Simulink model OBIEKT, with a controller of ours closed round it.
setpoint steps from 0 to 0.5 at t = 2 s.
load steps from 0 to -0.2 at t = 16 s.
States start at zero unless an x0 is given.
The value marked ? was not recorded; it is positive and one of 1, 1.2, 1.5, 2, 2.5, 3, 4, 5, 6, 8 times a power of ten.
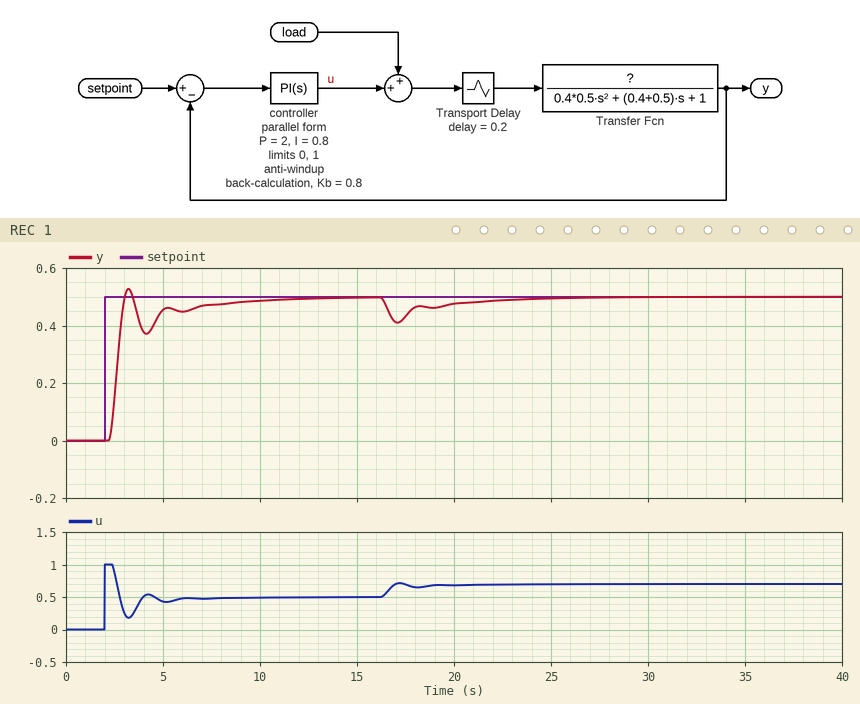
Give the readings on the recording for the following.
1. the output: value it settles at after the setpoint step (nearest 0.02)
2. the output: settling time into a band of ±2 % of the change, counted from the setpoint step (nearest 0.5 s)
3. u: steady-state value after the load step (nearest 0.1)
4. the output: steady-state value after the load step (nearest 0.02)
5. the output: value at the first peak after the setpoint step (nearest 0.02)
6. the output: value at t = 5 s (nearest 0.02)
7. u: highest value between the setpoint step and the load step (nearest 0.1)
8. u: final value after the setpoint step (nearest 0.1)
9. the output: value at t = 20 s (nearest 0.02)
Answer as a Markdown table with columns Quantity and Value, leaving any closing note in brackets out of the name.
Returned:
| Quantity | Value |
|---|---|
| the output: value it settles at after the setpoint step | 0.50 |
| the output: settling time into a band of ±2 % of the change, counted from the setpoint step | 9.0 s |
| u: steady-state value after the load step | 0.7 |
| the output: steady-state value after the load step | 0.50 |
| the output: value at the first peak after the setpoint step | 0.52 |
| the output: value at t = 5 s | 0.46 |
| u: highest value between the setpoint step and the load step | 1.0 |
| u: final value after the setpoint step | 0.5 |
| the output: value at t = 20 s | 0.48 |
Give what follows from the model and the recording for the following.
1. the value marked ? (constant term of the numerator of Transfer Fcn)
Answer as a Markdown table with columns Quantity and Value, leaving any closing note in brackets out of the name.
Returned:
| Quantity | Value |
|---|---|
| the value marked ? | 1 |
